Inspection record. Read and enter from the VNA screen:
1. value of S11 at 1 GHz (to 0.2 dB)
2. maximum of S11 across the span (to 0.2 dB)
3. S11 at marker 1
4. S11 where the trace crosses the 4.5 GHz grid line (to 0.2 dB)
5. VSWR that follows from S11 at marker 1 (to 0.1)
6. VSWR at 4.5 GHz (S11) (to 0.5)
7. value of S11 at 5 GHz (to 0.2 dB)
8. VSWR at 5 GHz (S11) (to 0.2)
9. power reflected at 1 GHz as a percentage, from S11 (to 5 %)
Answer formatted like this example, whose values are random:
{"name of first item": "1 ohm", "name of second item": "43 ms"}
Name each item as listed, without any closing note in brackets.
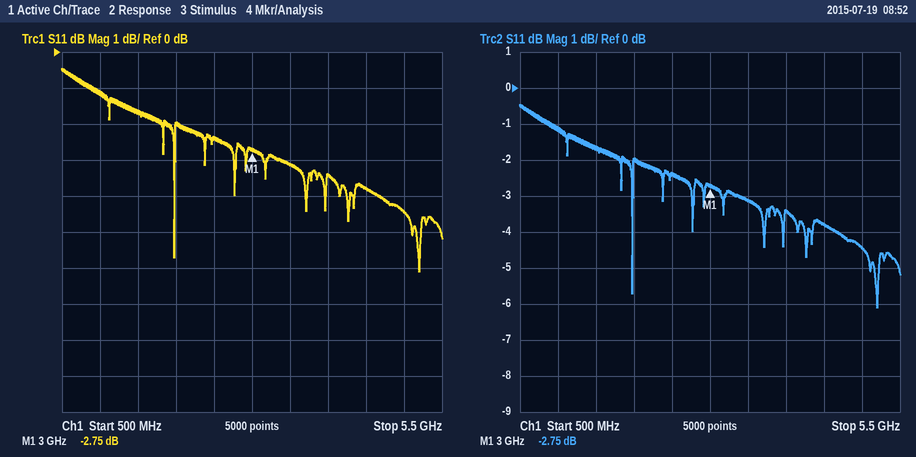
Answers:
{"value of S11 at 1 GHz": "-1.2 dB", "maximum of S11 across the span": "-0.4 dB", "S11 at marker 1": "-2.75 dB", "S11 where the trace crosses the 4.5 GHz grid line": "-3.8 dB", "VSWR that follows from S11 at marker 1": "6.4", "VSWR at 4.5 GHz (S11)": "4.5", "value of S11 at 5 GHz": "-4.4 dB", "VSWR at 5 GHz (S11)": "4.0", "power reflected at 1 GHz as a percentage, from S11": "75 %"}
